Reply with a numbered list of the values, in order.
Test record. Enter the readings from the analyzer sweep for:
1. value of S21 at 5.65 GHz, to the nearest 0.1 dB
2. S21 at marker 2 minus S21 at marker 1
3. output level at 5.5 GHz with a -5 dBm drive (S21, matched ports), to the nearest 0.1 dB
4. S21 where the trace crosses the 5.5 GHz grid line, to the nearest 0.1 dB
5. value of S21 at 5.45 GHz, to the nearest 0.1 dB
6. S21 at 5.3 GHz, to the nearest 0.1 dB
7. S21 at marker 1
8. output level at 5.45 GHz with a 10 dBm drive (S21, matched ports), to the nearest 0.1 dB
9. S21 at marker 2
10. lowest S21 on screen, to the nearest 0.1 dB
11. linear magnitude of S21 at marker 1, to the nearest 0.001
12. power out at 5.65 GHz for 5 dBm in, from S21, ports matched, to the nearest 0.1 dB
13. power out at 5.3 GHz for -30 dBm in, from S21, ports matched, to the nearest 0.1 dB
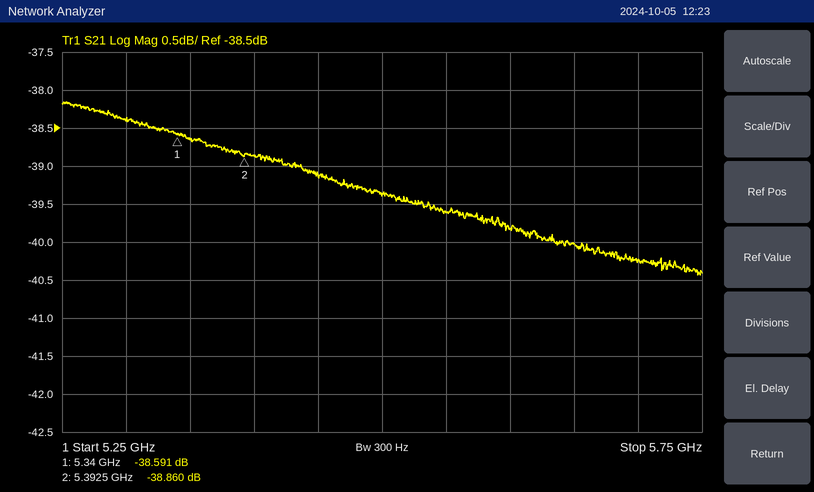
1. -40.0 dB
2. -0.269 dB
3. -44.4 dBm
4. -39.4 dB
5. -39.1 dB
6. -38.4 dB
7. -38.591 dB
8. -29.1 dBm
9. -38.860 dB
10. -40.4 dB
11. 0.012
12. -35.0 dBm
13. -68.4 dBm
